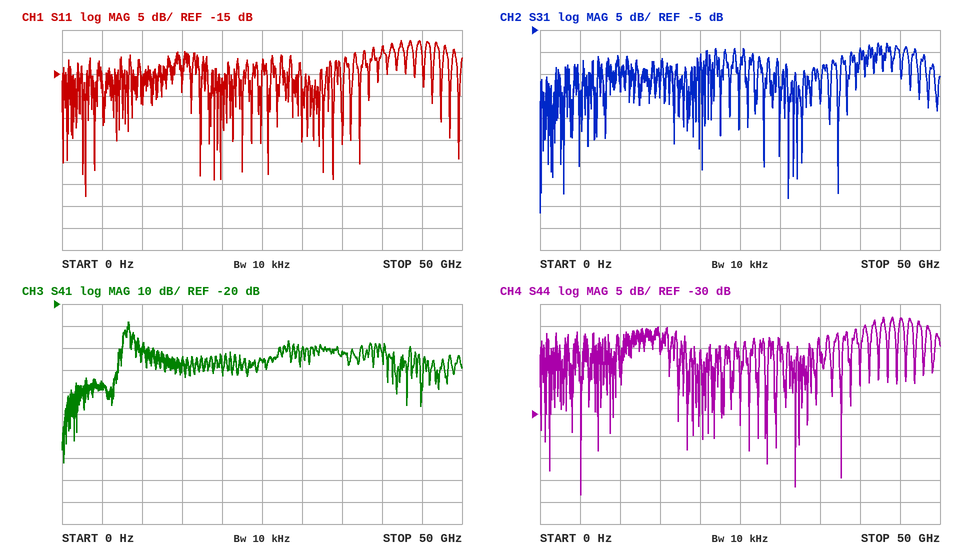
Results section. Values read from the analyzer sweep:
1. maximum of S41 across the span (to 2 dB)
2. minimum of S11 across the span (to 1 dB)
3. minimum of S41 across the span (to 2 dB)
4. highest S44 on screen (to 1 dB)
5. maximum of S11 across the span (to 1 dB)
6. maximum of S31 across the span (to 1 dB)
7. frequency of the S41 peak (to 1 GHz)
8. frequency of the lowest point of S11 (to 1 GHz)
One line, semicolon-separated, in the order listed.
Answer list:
-28 dB; -43 dB; -92 dB; -8 dB; -7 dB; -8 dB; 8 GHz; 3 GHz
